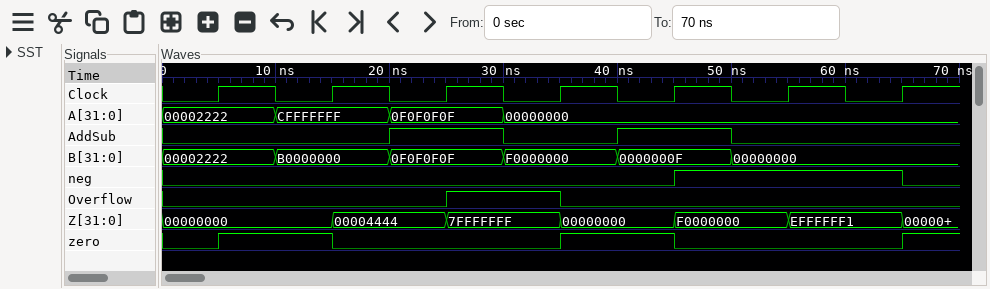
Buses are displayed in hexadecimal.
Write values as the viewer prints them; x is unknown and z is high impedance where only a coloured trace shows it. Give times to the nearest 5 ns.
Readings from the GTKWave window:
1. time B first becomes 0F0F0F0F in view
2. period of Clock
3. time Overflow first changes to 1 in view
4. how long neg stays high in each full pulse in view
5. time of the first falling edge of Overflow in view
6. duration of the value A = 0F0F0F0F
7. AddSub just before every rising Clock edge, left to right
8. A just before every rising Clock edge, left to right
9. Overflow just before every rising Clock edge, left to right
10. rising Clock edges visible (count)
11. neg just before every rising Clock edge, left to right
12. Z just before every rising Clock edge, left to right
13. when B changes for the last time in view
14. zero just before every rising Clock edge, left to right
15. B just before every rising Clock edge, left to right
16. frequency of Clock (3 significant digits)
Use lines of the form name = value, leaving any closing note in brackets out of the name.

time B first becomes 0F0F0F0F in view = 20 ns
period of Clock = 10 ns
time Overflow first changes to 1 in view = 25 ns
how long neg stays high in each full pulse in view = 20 ns
time of the first falling edge of Overflow in view = 35 ns
duration of the value A = 0F0F0F0F = 10 ns
AddSub just before every rising Clock edge, left to right = 0 0 1 0 1 0 0
A just before every rising Clock edge, left to right = 00002222, CFFFFFFF, 0F0F0F0F, 00000000, 00000000, 00000000, 00000000
Overflow just before every rising Clock edge, left to right = 0 0 0 1 0 0 0
rising Clock edges visible = 7
neg just before every rising Clock edge, left to right = 0 0 0 0 0 1 1
Z just before every rising Clock edge, left to right = 00000000, 00000000, 00004444, 7FFFFFFF, 00000000, F0000000, EFFFFFF1
when B changes for the last time in view = 50 ns
zero just before every rising Clock edge, left to right = 0 1 0 0 1 0 0
B just before every rising Clock edge, left to right = 00002222, B0000000, 0F0F0F0F, F0000000, 0000000F, 00000000, 00000000
frequency of Clock = 100 MHz
